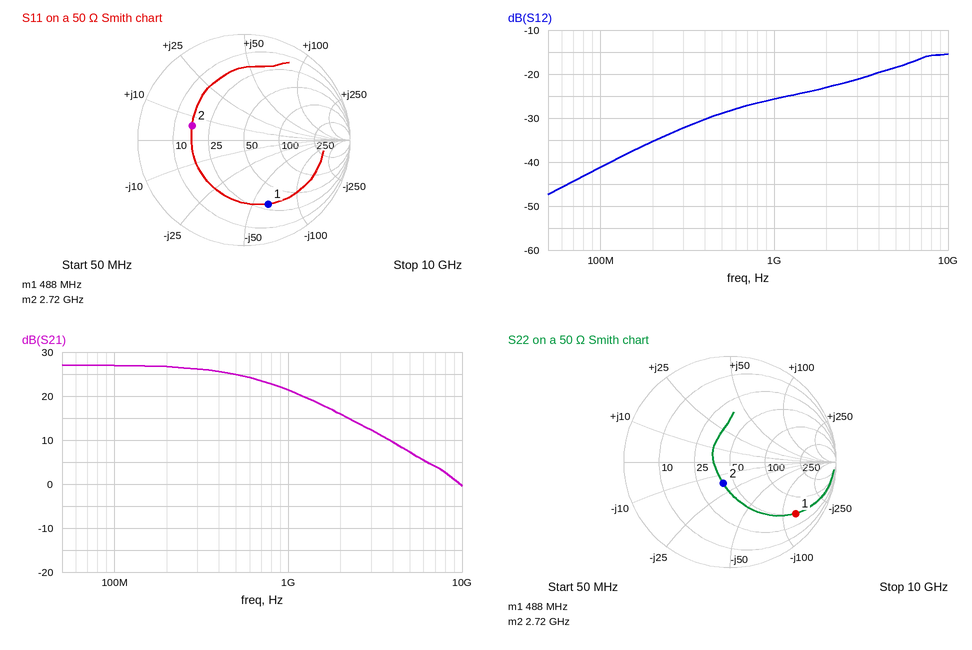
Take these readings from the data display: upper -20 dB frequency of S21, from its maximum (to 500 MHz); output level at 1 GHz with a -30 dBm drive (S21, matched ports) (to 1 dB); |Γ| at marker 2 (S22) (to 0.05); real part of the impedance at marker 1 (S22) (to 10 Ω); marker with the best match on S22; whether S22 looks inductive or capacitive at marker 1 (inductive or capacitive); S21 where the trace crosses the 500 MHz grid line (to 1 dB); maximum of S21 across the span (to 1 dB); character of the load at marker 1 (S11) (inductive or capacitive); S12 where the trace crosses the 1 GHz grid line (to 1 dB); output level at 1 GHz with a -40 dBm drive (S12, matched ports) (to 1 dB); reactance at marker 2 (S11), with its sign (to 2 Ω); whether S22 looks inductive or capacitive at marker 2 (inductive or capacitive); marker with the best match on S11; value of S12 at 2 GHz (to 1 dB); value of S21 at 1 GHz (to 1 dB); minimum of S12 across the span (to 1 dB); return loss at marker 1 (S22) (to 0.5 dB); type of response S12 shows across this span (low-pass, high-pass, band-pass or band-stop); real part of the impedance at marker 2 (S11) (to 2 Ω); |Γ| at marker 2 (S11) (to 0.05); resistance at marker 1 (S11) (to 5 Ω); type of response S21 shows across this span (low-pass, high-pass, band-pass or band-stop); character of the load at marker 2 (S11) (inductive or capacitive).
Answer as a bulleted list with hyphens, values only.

- 5.0 GHz
- -9 dBm
- 0.20
- 50 Ω
- marker 2
- capacitive
- 25 dB
- 27 dB
- capacitive
- -26 dB
- -66 dBm
- +6 Ω
- capacitive
- marker 2
- -23 dB
- 21 dB
- -47 dB
- 2.0 dB
- high-pass
- 16 Ω
- 0.50
- 30 Ω
- low-pass
- inductive
